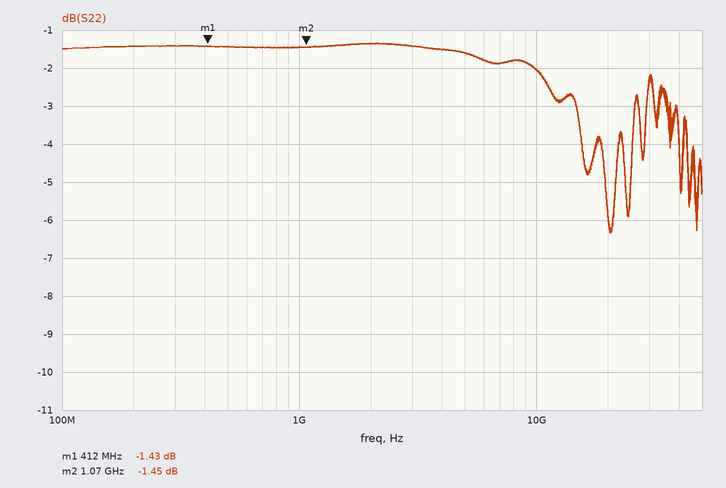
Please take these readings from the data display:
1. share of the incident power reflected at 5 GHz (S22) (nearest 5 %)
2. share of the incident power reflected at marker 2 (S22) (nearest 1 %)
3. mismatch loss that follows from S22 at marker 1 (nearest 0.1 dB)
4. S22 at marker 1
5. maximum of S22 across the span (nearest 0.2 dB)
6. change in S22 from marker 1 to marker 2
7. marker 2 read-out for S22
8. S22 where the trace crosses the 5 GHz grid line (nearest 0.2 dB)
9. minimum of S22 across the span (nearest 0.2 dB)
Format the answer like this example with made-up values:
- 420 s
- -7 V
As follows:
- 70 %
- 72 %
- 5.5 dB
- -1.43 dB
- -1.4 dB
- -0.02 dB
- -1.45 dB
- -1.6 dB
- -6.4 dB
